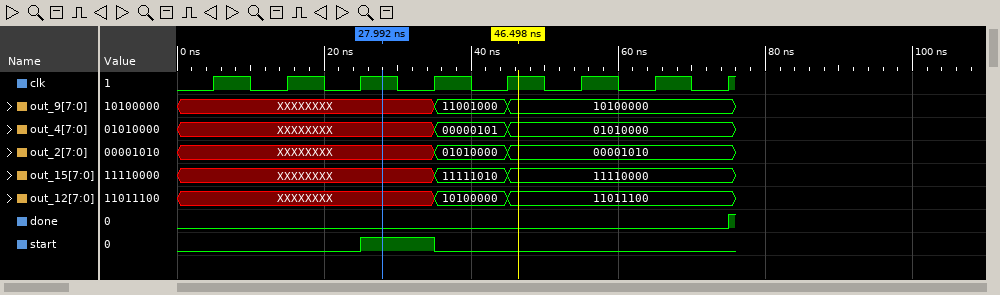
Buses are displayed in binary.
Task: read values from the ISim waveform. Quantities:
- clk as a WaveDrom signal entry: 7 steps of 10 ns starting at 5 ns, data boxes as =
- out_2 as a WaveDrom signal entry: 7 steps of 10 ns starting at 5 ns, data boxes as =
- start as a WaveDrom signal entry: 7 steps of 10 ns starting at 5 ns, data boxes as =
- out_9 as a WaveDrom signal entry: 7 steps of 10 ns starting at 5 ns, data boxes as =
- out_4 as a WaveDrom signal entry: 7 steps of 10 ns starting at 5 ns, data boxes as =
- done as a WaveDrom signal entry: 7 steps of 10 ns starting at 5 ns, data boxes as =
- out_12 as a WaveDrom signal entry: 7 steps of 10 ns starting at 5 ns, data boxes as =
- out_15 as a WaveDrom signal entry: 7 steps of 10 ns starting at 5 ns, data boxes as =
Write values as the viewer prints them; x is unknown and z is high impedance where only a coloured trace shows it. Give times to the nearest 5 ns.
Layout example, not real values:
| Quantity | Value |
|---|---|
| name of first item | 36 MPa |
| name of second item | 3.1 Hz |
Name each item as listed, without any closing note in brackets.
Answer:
| Quantity | Value |
|---|---|
| clk as a WaveDrom signal entry: 7 steps of 10 ns starting at 5 ns, data boxes as = | {name: 'clk', wave: 'p......'} |
| out_2 as a WaveDrom signal entry: 7 steps of 10 ns starting at 5 ns, data boxes as = | {name: 'out_2', wave: 'x..==..', data: '01010000 00001010'} |
| start as a WaveDrom signal entry: 7 steps of 10 ns starting at 5 ns, data boxes as = | {name: 'start', wave: '0.10...'} |
| out_9 as a WaveDrom signal entry: 7 steps of 10 ns starting at 5 ns, data boxes as = | {name: 'out_9', wave: 'x..==..', data: '11001000 10100000'} |
| out_4 as a WaveDrom signal entry: 7 steps of 10 ns starting at 5 ns, data boxes as = | {name: 'out_4', wave: 'x..==..', data: '00000101 01010000'} |
| done as a WaveDrom signal entry: 7 steps of 10 ns starting at 5 ns, data boxes as = | {name: 'done', wave: '0......'} |
| out_12 as a WaveDrom signal entry: 7 steps of 10 ns starting at 5 ns, data boxes as = | {name: 'out_12', wave: 'x..==..', data: '10100000 11011100'} |
| out_15 as a WaveDrom signal entry: 7 steps of 10 ns starting at 5 ns, data boxes as = | {name: 'out_15', wave: 'x..==..', data: '11111010 11110000'} |
